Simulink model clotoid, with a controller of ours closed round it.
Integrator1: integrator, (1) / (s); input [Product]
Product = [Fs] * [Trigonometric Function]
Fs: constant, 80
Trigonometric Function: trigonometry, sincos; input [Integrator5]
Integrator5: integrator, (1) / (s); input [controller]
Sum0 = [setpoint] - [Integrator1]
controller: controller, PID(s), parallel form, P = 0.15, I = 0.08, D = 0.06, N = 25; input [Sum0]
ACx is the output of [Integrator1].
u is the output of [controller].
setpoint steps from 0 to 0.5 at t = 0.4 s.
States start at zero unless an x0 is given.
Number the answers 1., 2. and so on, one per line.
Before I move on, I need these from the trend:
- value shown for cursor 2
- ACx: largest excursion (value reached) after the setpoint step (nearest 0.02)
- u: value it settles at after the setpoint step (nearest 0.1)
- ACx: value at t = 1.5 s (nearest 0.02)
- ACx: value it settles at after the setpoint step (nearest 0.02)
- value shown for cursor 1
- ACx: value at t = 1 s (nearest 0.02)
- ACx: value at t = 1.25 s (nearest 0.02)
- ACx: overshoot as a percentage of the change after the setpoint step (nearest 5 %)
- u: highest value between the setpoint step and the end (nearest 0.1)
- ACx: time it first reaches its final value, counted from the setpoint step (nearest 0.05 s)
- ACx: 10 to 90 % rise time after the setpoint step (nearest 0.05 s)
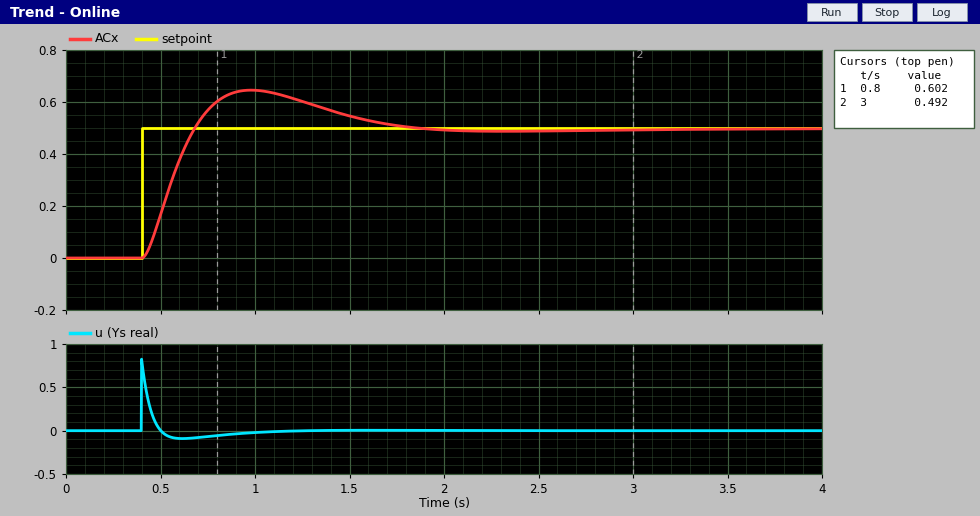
1. 0.492
2. 0.64
3. 0.0
4. 0.54
5. 0.50
6. 0.602
7. 0.64
8. 0.60
9. 30 %
10. 0.8
11. 0.30 s
12. 0.20 s
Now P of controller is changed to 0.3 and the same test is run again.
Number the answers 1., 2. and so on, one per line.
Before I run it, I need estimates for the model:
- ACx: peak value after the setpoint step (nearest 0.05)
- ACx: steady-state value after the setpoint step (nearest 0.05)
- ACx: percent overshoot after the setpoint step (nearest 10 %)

1. 0.70
2. 0.50
3. 40 %
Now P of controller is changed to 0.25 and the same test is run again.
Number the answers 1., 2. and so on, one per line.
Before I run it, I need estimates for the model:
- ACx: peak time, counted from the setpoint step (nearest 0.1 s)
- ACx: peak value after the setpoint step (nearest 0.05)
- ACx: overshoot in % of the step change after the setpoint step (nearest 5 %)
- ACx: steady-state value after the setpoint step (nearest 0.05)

1. 0.5 s
2. 0.70
3. 35 %
4. 0.50
